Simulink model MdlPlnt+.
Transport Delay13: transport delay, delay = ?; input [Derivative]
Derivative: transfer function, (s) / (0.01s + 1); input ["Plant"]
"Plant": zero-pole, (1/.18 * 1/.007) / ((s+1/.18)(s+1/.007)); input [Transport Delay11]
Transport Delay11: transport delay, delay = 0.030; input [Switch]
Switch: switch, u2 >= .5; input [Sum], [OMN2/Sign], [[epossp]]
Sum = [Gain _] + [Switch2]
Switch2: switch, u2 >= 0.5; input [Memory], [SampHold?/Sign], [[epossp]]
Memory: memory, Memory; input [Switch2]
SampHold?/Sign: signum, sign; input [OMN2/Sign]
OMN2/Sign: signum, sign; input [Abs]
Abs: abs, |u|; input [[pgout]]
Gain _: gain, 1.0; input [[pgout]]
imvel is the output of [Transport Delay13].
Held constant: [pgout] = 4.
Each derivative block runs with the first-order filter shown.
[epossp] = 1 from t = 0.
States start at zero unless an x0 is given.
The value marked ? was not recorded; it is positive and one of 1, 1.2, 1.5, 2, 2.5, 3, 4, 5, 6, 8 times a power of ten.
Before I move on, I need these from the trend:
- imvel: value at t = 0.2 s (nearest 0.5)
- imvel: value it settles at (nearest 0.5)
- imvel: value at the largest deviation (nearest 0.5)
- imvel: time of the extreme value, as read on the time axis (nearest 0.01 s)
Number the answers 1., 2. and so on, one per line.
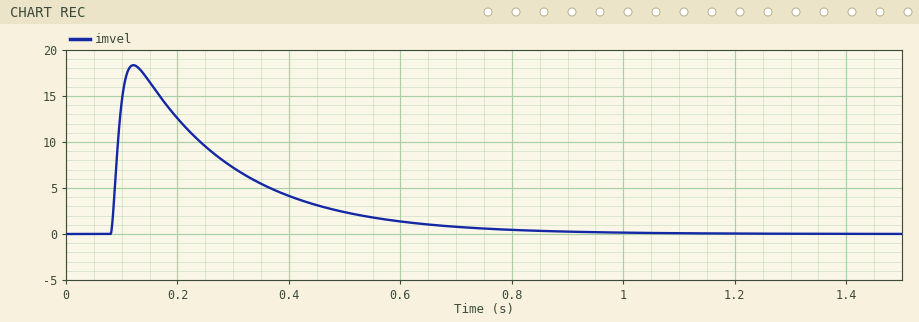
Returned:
1. 12.5
2. 0.0
3. 18.5
4. 0.12 s
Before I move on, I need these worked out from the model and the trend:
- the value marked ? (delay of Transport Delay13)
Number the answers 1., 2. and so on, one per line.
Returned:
1. 0.05
